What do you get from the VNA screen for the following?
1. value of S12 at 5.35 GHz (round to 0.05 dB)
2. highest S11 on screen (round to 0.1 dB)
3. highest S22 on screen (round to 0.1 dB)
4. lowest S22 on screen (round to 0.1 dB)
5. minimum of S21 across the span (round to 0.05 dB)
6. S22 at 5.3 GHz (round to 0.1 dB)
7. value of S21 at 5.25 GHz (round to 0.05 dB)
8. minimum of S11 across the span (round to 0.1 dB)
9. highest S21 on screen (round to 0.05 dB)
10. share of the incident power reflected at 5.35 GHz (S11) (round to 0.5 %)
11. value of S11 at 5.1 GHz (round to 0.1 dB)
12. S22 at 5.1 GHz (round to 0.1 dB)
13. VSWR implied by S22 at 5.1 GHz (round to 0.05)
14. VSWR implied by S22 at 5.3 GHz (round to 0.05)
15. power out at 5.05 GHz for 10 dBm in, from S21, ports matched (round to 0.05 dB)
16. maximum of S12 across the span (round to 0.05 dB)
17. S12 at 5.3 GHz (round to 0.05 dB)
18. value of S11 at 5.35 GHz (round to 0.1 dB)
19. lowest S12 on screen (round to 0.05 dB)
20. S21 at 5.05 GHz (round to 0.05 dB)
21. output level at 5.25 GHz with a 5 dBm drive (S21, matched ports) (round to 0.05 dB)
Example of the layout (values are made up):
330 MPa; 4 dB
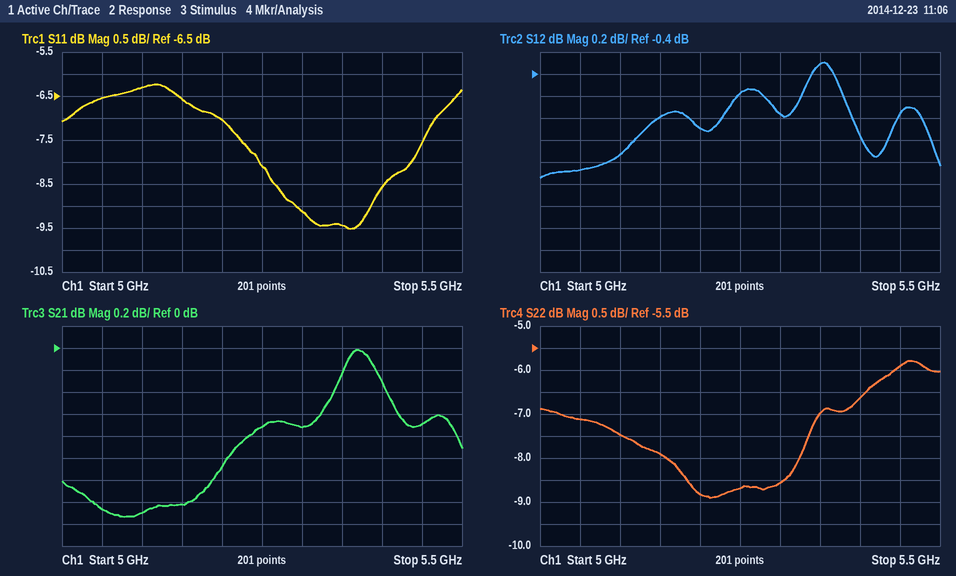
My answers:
-0.30 dB; -6.2 dB; -5.8 dB; -8.9 dB; -1.55 dB; -8.6 dB; -0.70 dB; -9.5 dB; 0.00 dB; 11.5 %; -6.3 dB; -7.5 dB; 2.45; 2.20; 8.55 dBm; -0.30 dB; -0.75 dB; -9.4 dB; -1.35 dB; -1.45 dB; 4.30 dBm
